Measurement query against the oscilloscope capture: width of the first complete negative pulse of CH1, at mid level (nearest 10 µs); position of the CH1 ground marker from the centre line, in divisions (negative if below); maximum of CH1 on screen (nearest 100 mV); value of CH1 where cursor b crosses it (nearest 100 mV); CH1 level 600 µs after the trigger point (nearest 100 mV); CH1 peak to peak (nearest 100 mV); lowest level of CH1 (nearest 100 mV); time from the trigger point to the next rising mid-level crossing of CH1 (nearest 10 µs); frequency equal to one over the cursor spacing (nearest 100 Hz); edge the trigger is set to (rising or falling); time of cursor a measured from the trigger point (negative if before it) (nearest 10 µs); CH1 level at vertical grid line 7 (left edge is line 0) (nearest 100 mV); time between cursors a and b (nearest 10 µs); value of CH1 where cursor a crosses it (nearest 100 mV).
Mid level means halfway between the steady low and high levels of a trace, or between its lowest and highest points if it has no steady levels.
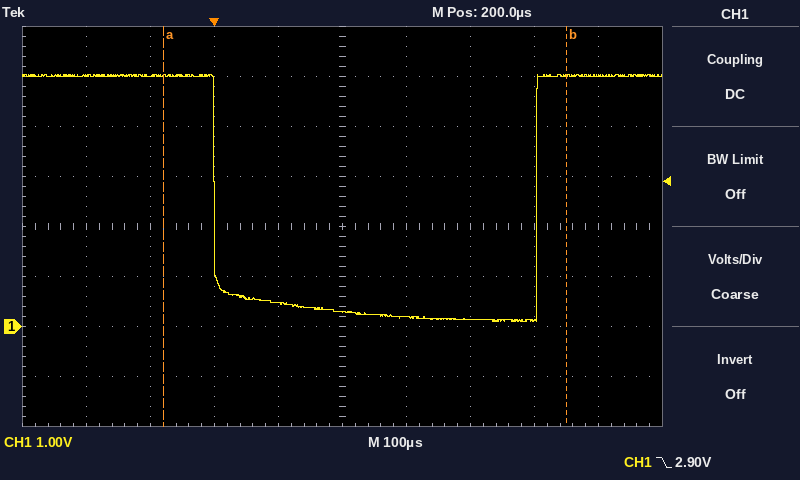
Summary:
500 µs
-2.0 div
5.0 V
5.0 V
5.0 V
4.9 V
100 mV
500 µs
1.6 kHz
falling
-80 µs
100 mV
630 µs
5.0 V
